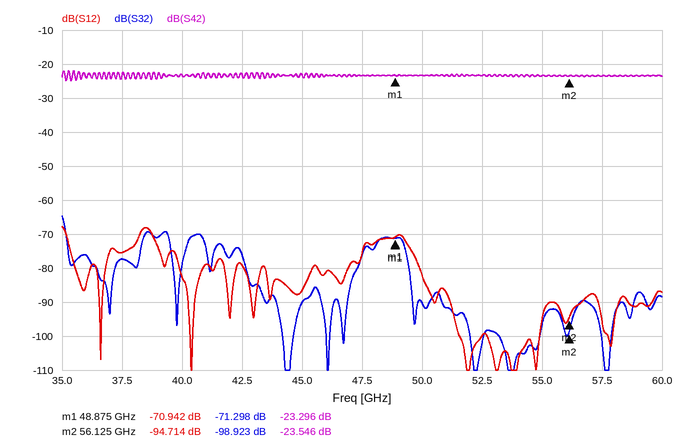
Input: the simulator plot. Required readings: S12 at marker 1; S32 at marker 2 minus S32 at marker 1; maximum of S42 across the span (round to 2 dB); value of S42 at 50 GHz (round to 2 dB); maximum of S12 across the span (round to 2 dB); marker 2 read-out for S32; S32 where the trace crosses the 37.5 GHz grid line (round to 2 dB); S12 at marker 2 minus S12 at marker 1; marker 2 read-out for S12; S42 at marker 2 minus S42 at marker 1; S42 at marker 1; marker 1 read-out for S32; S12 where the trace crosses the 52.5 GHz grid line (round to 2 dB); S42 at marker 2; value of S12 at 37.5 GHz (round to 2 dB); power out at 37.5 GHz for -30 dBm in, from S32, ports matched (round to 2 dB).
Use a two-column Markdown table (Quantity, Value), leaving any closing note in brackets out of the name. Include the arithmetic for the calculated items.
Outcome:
| Quantity | Value |
|---|---|
| S12 at marker 1 | -70.942 dB |
| S32 at marker 2 minus S32 at marker 1 | -98.923 − (-71.298) = -27.625 dB |
| maximum of S42 across the span | -22 dB |
| value of S42 at 50 GHz | -24 dB |
| maximum of S12 across the span | -68 dB |
| marker 2 read-out for S32 | -98.923 dB |
| S32 where the trace crosses the 37.5 GHz grid line | -78 dB |
| S12 at marker 2 minus S12 at marker 1 | -94.714 − (-70.942) = -23.772 dB |
| marker 2 read-out for S12 | -94.714 dB |
| S42 at marker 2 minus S42 at marker 1 | -23.546 − (-23.296) = -0.250 dB |
| S42 at marker 1 | -23.296 dB |
| marker 1 read-out for S32 | -71.298 dB |
| S12 where the trace crosses the 52.5 GHz grid line | -100 dB |
| S42 at marker 2 | -23.546 dB |
| value of S12 at 37.5 GHz | -76 dB |
| power out at 37.5 GHz for -30 dBm in, from S32, ports matched | -30 dBm + (-78 dB) = -108 dBm |
